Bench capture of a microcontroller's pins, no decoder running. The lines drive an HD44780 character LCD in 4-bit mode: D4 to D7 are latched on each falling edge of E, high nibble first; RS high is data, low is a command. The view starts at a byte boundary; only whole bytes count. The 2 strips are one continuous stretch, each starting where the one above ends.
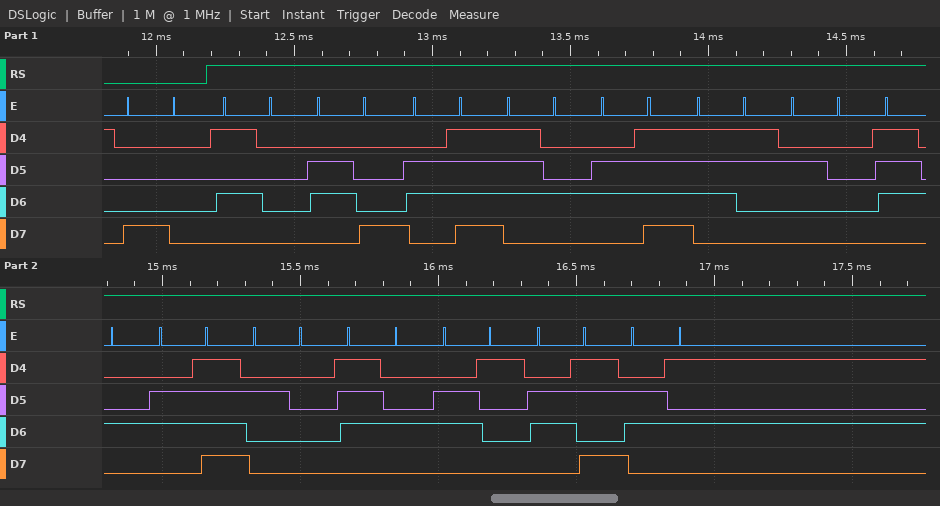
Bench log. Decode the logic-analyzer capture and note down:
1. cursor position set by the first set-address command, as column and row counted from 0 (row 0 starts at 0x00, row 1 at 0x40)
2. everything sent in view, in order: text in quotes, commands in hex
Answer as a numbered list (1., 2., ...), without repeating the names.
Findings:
1. column 0, row 0
2. 0x80 "Photos to take"
